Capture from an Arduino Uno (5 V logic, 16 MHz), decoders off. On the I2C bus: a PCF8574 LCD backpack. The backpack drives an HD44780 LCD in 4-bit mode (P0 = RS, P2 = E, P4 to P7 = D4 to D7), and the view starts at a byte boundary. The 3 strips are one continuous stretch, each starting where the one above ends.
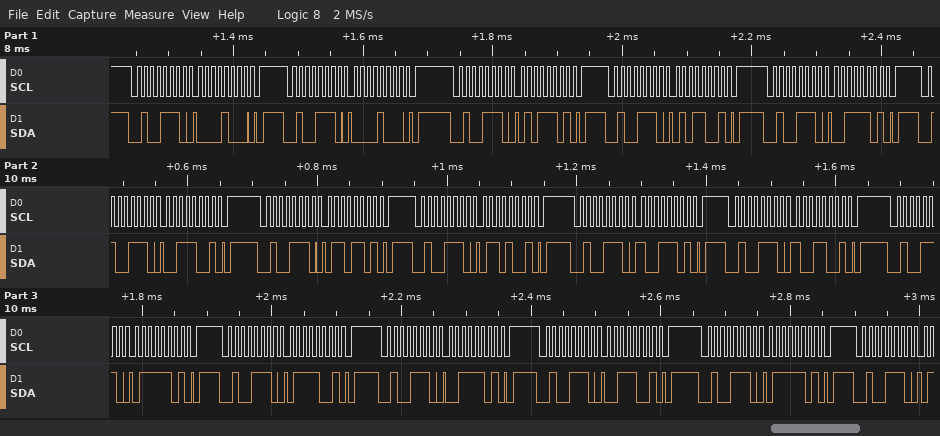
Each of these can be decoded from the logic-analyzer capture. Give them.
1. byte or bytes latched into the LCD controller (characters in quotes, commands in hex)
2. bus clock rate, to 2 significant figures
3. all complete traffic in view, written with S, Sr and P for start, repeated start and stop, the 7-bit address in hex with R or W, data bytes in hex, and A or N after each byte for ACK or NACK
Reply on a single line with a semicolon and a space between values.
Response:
'S' 'i' 's'; 100 kHz; S 27W A 08 A P S 27W A 08 A P S 27W A 5D A P S 27W A 59 A P S 27W A 3D A P S 27W A 39 A P S 27W A 6D A P S 27W A 69 A P S 27W A 9D A P S 27W A 99 A P S 27W A 7D A P S 27W A 79 A P S 27W A 3D A P S 27W A 39 A P S 27W A 7D A P S 27W A
